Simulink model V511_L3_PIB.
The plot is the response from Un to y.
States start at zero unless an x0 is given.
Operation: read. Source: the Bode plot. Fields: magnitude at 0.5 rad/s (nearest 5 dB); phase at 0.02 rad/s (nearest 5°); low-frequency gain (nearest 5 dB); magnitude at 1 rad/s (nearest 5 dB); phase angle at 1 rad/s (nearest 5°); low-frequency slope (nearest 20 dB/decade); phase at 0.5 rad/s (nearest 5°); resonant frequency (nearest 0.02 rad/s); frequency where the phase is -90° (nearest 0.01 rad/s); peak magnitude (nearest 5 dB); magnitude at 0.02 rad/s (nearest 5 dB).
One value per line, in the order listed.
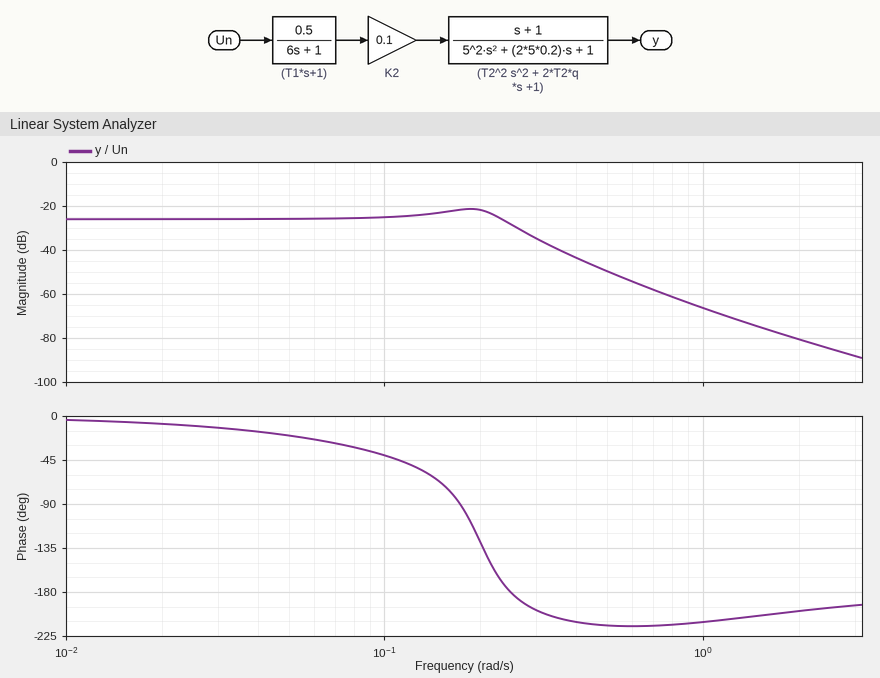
-50 dB
-10°
-25 dB
-65 dB
-210°
0 dB/decade
-215°
0.18 rad/s
0.17 rad/s
-20 dB
-25 dB
